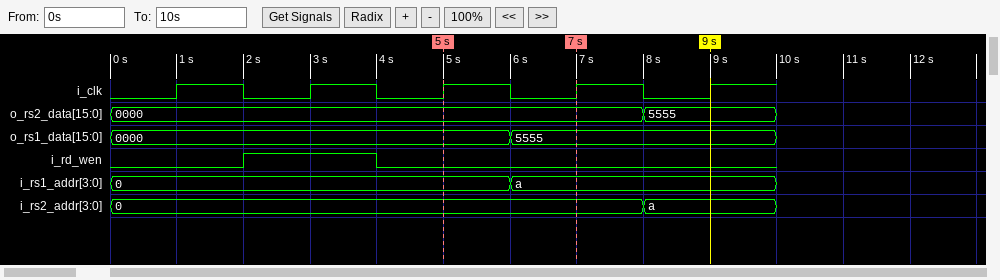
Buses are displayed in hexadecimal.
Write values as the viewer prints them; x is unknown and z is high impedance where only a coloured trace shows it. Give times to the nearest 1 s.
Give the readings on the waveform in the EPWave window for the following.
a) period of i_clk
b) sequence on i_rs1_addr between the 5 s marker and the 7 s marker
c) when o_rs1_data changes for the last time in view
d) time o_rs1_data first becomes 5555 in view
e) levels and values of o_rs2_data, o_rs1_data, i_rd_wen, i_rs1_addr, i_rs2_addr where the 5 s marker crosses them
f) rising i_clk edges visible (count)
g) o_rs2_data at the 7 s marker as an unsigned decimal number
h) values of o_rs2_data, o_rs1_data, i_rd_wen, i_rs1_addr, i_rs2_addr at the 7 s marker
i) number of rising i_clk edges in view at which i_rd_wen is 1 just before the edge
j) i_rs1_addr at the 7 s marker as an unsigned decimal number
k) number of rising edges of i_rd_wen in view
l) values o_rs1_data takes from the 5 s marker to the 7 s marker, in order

2 s
0, a
6 s
6 s
o_rs2_data=0000, o_rs1_data=0000, i_rd_wen=0, i_rs1_addr=0, i_rs2_addr=0
5
0
o_rs2_data=0000, o_rs1_data=5555, i_rd_wen=0, i_rs1_addr=a, i_rs2_addr=0
1
10
1
0000, 5555
